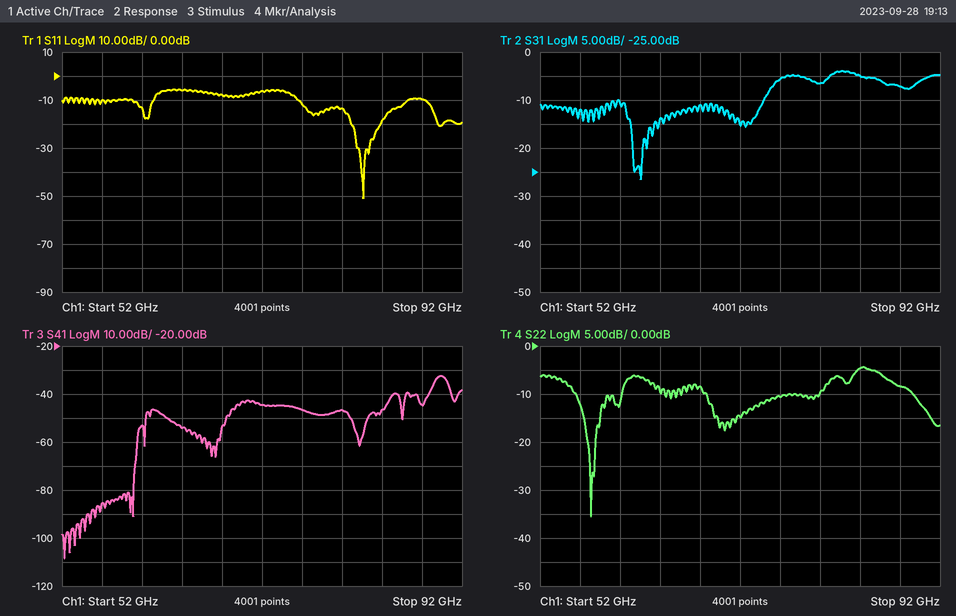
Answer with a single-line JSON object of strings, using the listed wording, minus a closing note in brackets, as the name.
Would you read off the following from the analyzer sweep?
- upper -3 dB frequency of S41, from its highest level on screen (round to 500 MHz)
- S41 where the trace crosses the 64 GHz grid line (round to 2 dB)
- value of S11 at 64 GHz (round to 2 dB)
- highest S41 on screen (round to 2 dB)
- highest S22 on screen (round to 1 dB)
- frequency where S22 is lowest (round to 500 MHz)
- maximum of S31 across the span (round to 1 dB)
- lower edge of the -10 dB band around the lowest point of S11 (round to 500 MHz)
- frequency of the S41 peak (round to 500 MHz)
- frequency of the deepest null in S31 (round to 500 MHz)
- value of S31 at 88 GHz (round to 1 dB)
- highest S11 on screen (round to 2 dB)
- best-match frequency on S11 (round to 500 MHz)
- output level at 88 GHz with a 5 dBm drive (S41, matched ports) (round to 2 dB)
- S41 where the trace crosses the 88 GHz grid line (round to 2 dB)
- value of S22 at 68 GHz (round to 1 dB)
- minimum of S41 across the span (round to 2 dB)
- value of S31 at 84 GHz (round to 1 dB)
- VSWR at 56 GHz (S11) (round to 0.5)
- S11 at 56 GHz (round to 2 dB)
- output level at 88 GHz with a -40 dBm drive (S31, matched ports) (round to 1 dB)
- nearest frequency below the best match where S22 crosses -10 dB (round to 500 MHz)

{"upper -3 dB frequency of S41, from its highest level on screen": "90.5 GHz", "S41 where the trace crosses the 64 GHz grid line": "-54 dB", "value of S11 at 64 GHz": "-6 dB", "highest S41 on screen": "-32 dB", "highest S22 on screen": "-4 dB", "frequency where S22 is lowest": "57.0 GHz", "maximum of S31 across the span": "-4 dB", "lower edge of the -10 dB band around the lowest point of S11": "75.5 GHz", "frequency of the S41 peak": "90.0 GHz", "frequency of the deepest null in S31": "62.0 GHz", "value of S31 at 88 GHz": "-7 dB", "highest S11 on screen": "-6 dB", "best-match frequency on S11": "82.0 GHz", "output level at 88 GHz with a 5 dBm drive (S41, matched ports)": "-40 dBm", "S41 where the trace crosses the 88 GHz grid line": "-44 dB", "value of S22 at 68 GHz": "-8 dB", "minimum of S41 across the span": "-108 dB", "value of S31 at 84 GHz": "-5 dB", "VSWR at 56 GHz (S11)": "2.0", "S11 at 56 GHz": "-10 dB", "output level at 88 GHz with a -40 dBm drive (S31, matched ports)": "-47 dBm", "nearest frequency below the best match where S22 crosses -10 dB": "55.5 GHz"}
